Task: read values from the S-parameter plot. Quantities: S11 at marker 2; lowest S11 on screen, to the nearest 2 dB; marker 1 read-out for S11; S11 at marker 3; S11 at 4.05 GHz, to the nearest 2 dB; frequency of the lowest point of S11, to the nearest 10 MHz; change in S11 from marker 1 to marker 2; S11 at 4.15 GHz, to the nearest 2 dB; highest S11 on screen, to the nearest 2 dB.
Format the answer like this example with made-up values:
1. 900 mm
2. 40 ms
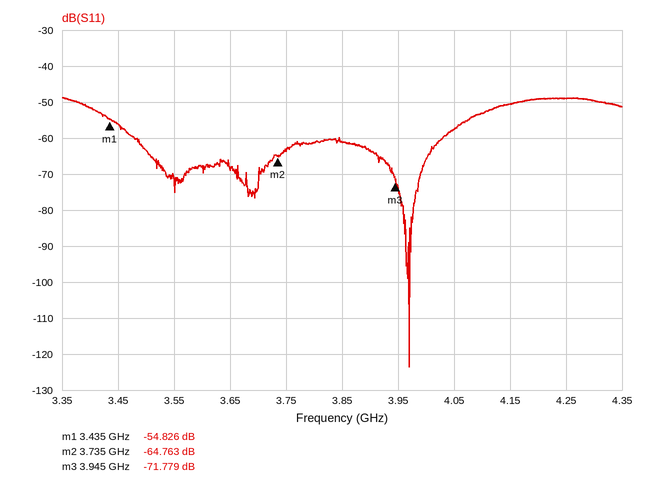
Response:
1. -64.763 dB
2. -124 dB
3. -54.826 dB
4. -71.779 dB
5. -58 dB
6. 3.97 GHz
7. -9.937 dB
8. -50 dB
9. -48 dB
